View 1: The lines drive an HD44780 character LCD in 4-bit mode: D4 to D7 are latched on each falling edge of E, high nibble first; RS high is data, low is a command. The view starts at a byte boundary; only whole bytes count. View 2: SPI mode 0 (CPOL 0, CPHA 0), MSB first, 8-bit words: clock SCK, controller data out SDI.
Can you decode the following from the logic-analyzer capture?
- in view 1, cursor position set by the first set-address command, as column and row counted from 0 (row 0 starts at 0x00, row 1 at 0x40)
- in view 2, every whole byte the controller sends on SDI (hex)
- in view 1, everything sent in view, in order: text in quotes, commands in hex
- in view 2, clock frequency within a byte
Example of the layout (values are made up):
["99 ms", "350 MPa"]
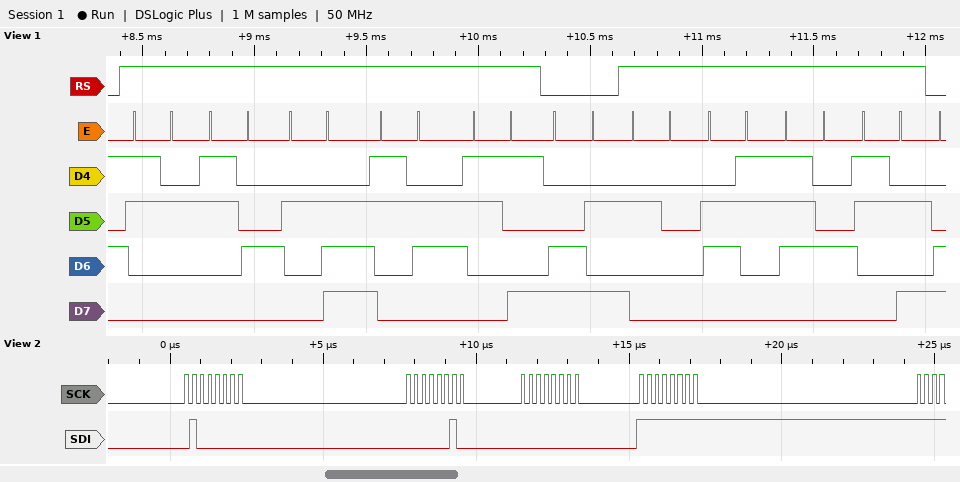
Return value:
["column 10, row 1", "40 02 00 FF", "\"24.69\" 0xCA \" ct:\"", "4 MHz"]
